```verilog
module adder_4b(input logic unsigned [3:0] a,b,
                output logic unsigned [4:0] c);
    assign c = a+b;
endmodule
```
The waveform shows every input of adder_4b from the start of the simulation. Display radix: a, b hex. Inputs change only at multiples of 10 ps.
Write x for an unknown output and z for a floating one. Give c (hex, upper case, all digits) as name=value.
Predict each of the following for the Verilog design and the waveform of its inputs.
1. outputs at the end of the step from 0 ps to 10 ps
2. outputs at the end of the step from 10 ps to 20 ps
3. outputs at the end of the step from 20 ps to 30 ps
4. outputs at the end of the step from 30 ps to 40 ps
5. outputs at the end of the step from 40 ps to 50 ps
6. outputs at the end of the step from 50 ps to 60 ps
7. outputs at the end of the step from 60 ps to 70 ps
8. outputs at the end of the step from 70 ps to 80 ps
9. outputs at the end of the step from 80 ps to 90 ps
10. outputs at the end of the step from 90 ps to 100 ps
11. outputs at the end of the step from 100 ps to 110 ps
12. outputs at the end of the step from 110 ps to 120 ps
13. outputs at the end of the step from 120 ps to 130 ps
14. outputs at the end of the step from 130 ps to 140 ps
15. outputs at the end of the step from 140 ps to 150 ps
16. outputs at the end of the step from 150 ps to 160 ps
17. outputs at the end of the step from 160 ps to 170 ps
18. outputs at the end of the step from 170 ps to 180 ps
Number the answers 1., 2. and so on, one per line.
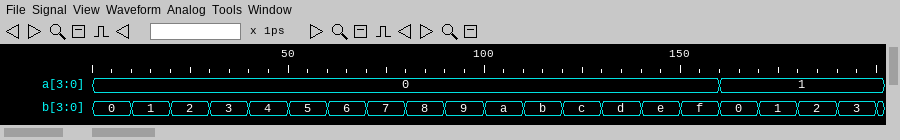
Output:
1. c=00
2. c=01
3. c=02
4. c=03
5. c=04
6. c=05
7. c=06
8. c=07
9. c=08
10. c=09
11. c=0A
12. c=0B
13. c=0C
14. c=0D
15. c=0E
16. c=0F
17. c=01
18. c=02
